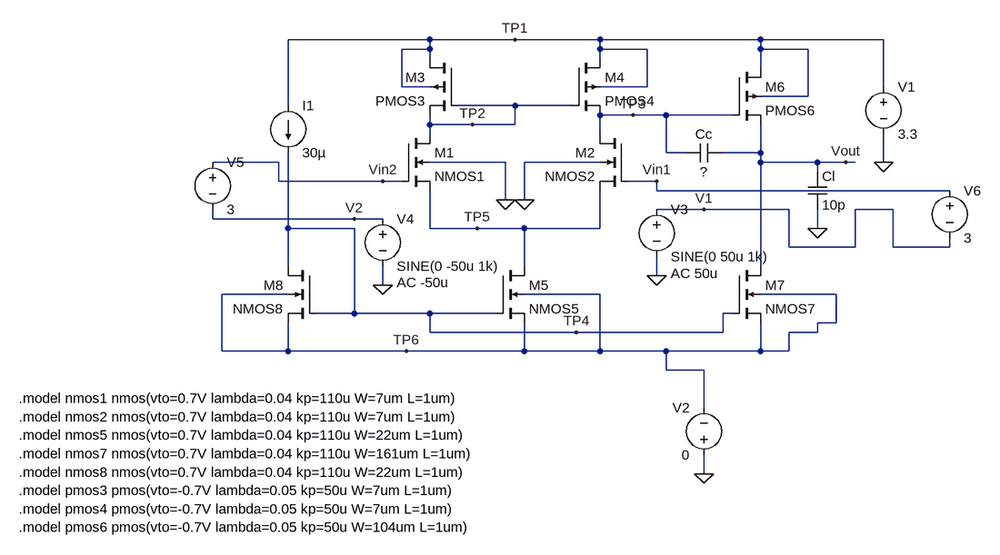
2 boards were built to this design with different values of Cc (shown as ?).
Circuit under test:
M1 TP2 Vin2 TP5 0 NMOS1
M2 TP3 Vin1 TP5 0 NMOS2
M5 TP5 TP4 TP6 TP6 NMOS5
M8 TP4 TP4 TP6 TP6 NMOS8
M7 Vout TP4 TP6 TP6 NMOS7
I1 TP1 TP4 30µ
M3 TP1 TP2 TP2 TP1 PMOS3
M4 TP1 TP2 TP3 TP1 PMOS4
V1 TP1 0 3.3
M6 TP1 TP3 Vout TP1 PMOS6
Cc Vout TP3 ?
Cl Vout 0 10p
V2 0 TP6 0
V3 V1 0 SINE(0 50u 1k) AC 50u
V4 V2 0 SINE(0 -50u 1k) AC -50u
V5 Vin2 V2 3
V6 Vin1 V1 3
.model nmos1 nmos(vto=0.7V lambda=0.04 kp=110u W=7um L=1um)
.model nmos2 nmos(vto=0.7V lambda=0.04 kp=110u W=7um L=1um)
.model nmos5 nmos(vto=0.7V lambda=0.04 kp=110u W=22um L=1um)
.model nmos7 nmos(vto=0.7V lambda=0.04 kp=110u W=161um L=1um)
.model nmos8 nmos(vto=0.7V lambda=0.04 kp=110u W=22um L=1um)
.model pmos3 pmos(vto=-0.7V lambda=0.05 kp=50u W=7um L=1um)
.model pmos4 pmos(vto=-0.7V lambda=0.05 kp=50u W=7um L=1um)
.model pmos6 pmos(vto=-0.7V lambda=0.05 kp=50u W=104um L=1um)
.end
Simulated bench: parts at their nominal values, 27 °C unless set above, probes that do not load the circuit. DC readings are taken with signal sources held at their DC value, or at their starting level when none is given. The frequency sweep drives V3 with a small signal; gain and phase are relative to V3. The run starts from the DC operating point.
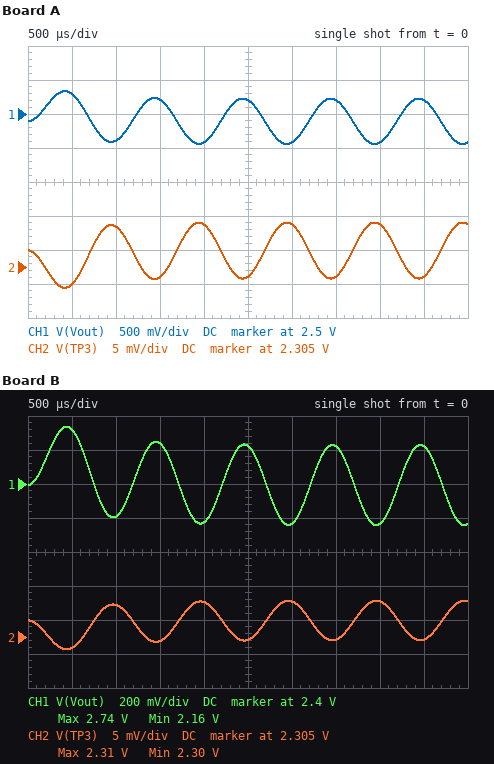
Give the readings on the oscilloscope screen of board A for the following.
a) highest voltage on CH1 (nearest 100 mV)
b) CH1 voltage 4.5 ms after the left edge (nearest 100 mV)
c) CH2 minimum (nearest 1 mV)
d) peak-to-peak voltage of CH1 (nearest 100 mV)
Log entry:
2.8 V
2.7 V
2.302 V
800 mV
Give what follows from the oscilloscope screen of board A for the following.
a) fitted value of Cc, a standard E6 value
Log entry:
6.8 pF
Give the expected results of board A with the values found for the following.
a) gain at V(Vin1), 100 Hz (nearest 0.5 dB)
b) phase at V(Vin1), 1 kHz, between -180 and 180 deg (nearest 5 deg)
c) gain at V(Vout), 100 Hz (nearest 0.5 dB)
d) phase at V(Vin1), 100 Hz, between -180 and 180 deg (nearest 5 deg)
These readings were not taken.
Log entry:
0 dB
0 deg
79.0 dB
0 deg
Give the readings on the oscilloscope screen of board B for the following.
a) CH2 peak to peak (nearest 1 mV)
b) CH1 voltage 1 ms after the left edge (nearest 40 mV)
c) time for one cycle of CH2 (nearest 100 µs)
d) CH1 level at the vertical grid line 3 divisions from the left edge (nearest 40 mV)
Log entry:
7 mV
2.20 V
1.0 ms
2.64 V
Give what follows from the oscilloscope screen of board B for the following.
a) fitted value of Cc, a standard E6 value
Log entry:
10 pF
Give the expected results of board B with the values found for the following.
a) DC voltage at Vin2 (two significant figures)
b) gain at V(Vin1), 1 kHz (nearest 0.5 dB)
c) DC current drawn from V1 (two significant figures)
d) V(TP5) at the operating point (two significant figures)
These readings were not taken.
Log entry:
3.0 V
0 dB
290 µA
2.1 V
